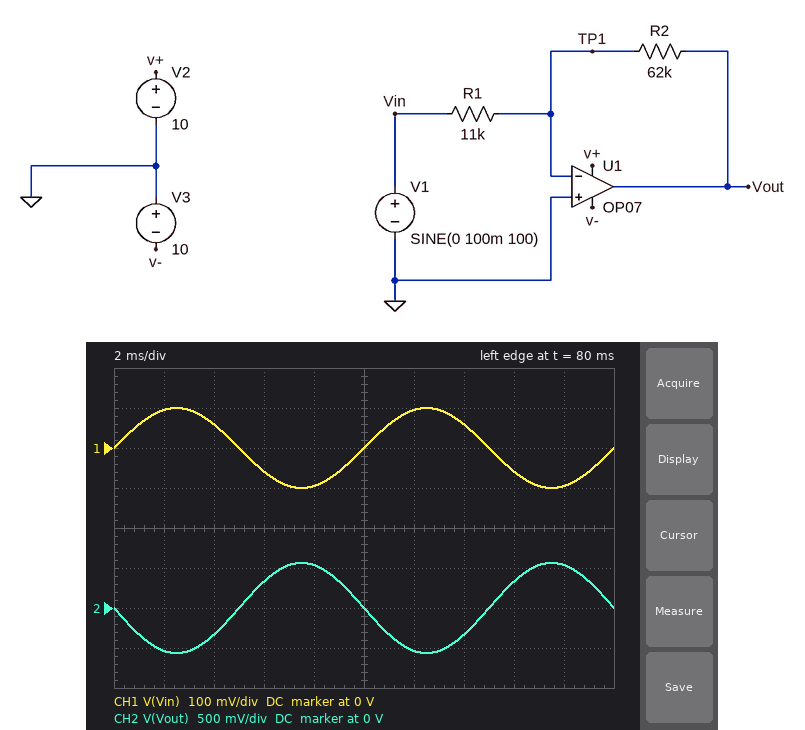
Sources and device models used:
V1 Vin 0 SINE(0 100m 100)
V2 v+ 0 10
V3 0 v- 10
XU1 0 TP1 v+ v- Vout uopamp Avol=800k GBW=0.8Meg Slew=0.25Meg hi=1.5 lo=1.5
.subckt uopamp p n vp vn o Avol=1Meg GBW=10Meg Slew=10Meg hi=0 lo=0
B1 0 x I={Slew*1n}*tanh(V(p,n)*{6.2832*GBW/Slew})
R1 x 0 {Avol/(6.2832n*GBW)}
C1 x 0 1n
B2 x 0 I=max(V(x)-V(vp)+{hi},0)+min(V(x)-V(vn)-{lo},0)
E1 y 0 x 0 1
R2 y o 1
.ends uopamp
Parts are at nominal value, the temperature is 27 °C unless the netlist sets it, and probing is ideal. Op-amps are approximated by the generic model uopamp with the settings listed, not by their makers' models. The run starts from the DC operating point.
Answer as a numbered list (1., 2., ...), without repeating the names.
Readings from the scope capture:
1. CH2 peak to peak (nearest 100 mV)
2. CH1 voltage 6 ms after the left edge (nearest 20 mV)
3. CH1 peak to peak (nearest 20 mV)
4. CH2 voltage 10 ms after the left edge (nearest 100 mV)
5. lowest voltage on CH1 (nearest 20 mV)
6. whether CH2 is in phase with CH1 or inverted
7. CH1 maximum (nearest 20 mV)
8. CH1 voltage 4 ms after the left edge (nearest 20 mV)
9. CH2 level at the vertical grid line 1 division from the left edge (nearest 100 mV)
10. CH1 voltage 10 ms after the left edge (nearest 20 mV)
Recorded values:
1. 1.1 V
2. -60 mV
3. 200 mV
4. 0 V
5. -100 mV
6. inverted
7. 100 mV
8. 60 mV
9. -500 mV
10. 0 V
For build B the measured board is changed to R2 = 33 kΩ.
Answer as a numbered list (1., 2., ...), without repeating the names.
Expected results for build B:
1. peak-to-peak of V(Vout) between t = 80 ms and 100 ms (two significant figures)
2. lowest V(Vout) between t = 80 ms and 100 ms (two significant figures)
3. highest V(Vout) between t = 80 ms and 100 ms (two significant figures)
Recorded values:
1. 600 mV
2. -300 mV
3. 300 mV
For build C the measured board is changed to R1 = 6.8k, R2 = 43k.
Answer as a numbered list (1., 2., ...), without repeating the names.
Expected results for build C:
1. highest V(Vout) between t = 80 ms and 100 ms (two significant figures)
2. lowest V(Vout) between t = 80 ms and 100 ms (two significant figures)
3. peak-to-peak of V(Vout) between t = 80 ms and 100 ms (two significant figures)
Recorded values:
1. 630 mV
2. -630 mV
3. 1.3 V
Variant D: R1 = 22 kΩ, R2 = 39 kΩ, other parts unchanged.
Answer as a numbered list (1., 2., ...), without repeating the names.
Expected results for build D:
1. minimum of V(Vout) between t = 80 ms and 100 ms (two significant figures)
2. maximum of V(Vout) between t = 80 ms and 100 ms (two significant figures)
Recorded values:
1. -180 mV
2. 180 mV
